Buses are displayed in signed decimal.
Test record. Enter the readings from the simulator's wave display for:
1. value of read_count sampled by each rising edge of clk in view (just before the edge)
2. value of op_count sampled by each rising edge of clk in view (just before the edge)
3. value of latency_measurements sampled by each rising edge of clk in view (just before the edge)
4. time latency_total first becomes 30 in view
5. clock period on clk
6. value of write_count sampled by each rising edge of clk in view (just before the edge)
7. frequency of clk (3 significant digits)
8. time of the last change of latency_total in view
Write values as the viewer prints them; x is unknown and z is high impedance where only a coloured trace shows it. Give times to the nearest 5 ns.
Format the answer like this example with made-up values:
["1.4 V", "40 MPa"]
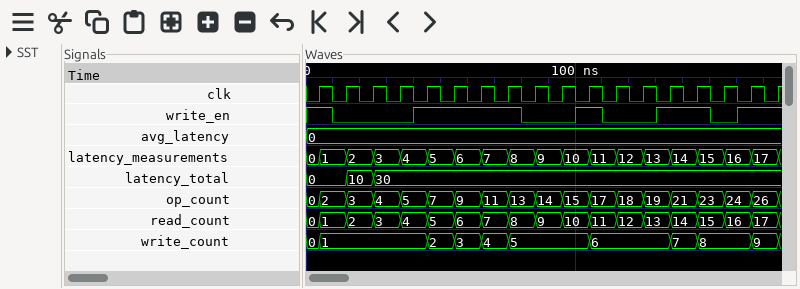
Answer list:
["0, 1, 2, 3, 4, 5, 6, 7, 8, 9, 10, 11, 12, 13, 14, 15, 16, 17", "0, 2, 3, 4, 5, 7, 9, 11, 13, 14, 15, 17, 18, 19, 21, 23, 24, 26", "0, 1, 2, 3, 4, 5, 6, 7, 8, 9, 10, 11, 12, 13, 14, 15, 16, 17", "25 ns", "10 ns", "0, 1, 1, 1, 1, 2, 3, 4, 5, 5, 5, 6, 6, 6, 7, 8, 8, 9", "100 MHz", "25 ns"]
